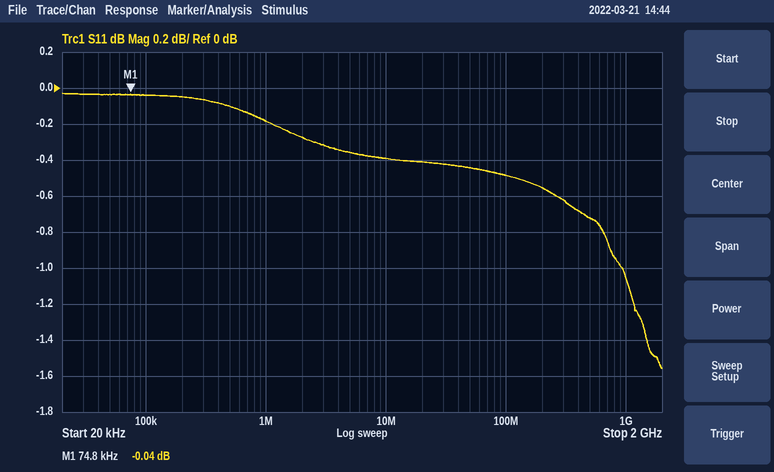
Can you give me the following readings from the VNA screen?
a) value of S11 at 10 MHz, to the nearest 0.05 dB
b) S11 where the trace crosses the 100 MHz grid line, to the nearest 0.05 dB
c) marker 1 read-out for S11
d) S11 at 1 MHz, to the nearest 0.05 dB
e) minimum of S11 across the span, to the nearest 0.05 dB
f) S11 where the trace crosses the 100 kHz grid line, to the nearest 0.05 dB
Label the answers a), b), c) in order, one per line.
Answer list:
a) -0.40 dB
b) -0.50 dB
c) -0.04 dB
d) -0.20 dB
e) -1.55 dB
f) -0.05 dB
